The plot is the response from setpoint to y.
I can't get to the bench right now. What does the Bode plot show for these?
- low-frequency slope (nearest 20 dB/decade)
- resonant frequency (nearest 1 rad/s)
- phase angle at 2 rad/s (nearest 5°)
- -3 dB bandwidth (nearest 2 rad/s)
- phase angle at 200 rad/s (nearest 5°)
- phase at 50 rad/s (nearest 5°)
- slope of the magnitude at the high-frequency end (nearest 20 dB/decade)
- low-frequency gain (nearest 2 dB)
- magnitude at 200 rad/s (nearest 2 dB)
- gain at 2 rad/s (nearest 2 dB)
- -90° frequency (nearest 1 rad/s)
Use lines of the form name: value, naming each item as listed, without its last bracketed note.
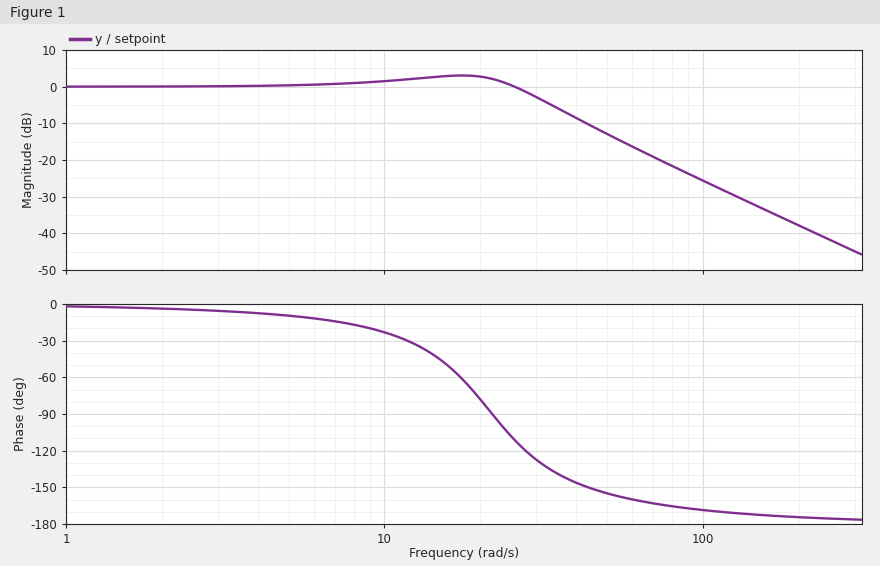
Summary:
low-frequency slope: 0 dB/decade
resonant frequency: 17 rad/s
phase angle at 2 rad/s: -5°
-3 dB bandwidth: 30 rad/s
phase angle at 200 rad/s: -175°
phase at 50 rad/s: -155°
slope of the magnitude at the high-frequency end: -40 dB/decade
low-frequency gain: 0 dB
magnitude at 200 rad/s: -38 dB
gain at 2 rad/s: 0 dB
-90° frequency: 22 rad/s
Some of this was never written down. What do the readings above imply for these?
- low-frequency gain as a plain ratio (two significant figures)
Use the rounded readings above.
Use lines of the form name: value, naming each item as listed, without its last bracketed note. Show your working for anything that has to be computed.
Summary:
low-frequency gain as a plain ratio: 10^(0 / 20) = 1.0
